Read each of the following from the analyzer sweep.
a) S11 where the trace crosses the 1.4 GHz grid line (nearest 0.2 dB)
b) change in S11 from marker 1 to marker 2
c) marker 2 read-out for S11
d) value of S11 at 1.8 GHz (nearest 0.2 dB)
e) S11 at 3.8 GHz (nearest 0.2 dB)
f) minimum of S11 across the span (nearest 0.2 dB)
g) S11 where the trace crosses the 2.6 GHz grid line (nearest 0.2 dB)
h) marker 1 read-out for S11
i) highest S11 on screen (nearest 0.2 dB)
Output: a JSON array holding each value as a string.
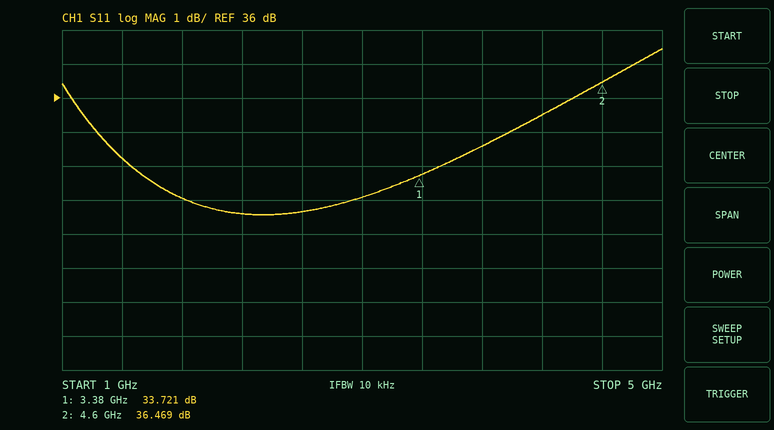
["34.2 dB", "2.748 dB", "36.469 dB", "33.0 dB", "34.6 dB", "32.6 dB", "32.6 dB", "33.721 dB", "37.4 dB"]
